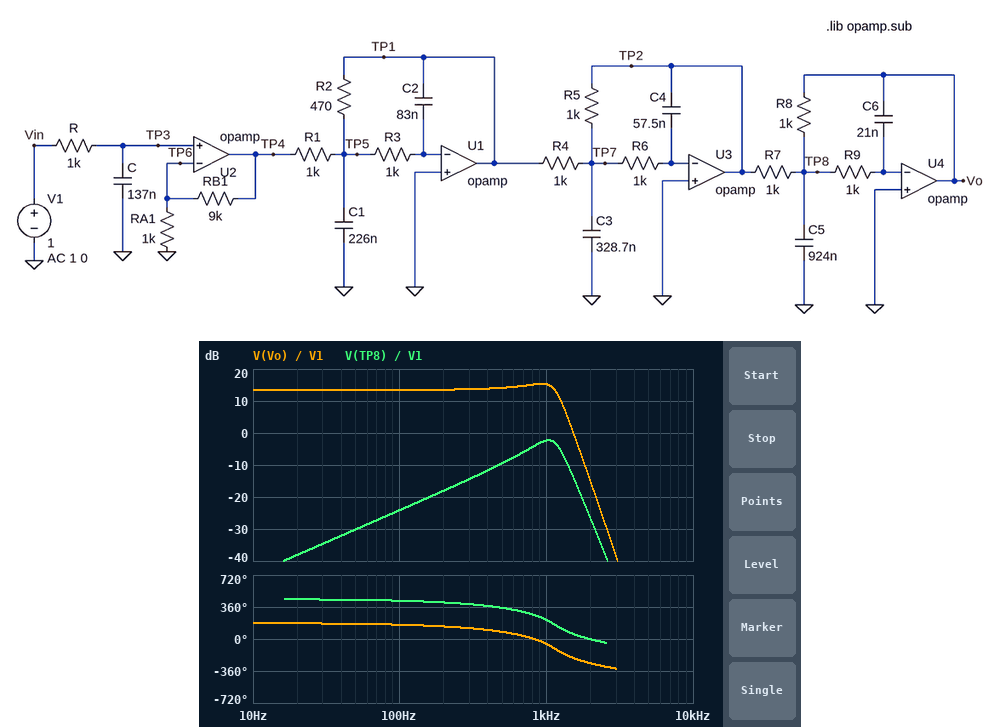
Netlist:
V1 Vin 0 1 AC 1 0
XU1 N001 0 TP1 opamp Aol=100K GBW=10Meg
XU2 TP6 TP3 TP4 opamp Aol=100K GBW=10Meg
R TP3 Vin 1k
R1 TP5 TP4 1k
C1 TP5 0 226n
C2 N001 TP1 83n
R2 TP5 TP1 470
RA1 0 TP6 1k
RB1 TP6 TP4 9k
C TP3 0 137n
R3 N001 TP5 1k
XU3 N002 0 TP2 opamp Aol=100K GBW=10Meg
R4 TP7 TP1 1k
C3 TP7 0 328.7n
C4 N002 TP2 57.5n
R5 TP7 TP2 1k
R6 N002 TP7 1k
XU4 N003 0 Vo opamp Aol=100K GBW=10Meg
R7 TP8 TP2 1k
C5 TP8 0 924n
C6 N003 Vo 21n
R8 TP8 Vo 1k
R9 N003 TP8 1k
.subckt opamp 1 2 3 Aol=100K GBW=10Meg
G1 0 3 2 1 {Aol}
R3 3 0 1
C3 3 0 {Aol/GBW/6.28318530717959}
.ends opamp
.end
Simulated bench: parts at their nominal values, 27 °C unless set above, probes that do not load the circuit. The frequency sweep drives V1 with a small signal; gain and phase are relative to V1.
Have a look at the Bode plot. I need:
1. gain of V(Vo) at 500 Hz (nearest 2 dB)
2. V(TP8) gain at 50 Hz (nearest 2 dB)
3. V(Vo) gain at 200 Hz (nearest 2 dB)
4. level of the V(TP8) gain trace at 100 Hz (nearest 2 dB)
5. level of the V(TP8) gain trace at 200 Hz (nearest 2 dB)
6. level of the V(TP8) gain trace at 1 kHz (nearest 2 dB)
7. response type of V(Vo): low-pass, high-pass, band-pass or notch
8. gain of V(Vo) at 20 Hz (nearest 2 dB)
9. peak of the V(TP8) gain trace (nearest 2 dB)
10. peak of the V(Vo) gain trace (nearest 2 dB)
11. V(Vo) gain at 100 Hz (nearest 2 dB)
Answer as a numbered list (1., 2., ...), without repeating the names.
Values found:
1. 14 dB
2. -30 dB
3. 14 dB
4. -24 dB
5. -18 dB
6. -2 dB
7. low-pass
8. 14 dB
9. -2 dB
10. 16 dB
11. 14 dB
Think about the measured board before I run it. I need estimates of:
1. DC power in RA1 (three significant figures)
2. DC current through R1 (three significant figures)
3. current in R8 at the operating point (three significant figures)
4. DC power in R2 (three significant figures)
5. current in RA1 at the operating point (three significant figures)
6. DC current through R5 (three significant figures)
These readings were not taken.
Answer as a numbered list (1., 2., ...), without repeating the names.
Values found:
1. 1.00 mW
2. 10.0 mA
3. 4.70 mA
4. 47.0 mW
5. 1.00 mA
6. 4.70 mA
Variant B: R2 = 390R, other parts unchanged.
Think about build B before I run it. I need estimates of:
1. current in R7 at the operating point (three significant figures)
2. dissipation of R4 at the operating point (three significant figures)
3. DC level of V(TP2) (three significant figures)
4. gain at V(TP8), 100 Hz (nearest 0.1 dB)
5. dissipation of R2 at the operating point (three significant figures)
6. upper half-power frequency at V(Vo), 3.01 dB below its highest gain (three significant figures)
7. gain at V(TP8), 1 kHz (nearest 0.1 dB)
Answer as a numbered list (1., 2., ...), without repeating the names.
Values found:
1. 3.90 mA
2. 15.2 mW
3. 3.90 V
4. -25.7 dB
5. 39.0 mW
6. 1.19 kHz
7. -3.7 dB
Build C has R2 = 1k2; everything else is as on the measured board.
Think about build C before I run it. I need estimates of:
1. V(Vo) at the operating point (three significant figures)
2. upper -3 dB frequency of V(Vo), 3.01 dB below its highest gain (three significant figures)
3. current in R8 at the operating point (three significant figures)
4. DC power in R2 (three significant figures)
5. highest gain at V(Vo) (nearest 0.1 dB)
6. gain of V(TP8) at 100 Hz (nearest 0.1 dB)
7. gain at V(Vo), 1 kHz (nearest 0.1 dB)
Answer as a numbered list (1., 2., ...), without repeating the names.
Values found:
1. -12.0 V
2. 1.10 kHz
3. 12.0 mA
4. 120 mW
5. 21.6 dB
6. -16.0 dB
7. 20.0 dB
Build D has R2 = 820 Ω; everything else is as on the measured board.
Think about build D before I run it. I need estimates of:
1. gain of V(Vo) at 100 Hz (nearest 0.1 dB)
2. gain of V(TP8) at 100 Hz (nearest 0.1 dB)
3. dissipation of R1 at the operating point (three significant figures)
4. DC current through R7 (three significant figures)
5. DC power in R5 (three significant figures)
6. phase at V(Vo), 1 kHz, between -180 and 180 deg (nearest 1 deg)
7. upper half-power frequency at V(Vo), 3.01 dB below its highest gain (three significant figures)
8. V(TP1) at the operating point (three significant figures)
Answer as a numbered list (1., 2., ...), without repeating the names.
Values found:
1. 18.3 dB
2. -19.3 dB
3. 100 mW
4. 8.20 mA
5. 67.2 mW
6. -71 deg
7. 1.16 kHz
8. -8.20 V
